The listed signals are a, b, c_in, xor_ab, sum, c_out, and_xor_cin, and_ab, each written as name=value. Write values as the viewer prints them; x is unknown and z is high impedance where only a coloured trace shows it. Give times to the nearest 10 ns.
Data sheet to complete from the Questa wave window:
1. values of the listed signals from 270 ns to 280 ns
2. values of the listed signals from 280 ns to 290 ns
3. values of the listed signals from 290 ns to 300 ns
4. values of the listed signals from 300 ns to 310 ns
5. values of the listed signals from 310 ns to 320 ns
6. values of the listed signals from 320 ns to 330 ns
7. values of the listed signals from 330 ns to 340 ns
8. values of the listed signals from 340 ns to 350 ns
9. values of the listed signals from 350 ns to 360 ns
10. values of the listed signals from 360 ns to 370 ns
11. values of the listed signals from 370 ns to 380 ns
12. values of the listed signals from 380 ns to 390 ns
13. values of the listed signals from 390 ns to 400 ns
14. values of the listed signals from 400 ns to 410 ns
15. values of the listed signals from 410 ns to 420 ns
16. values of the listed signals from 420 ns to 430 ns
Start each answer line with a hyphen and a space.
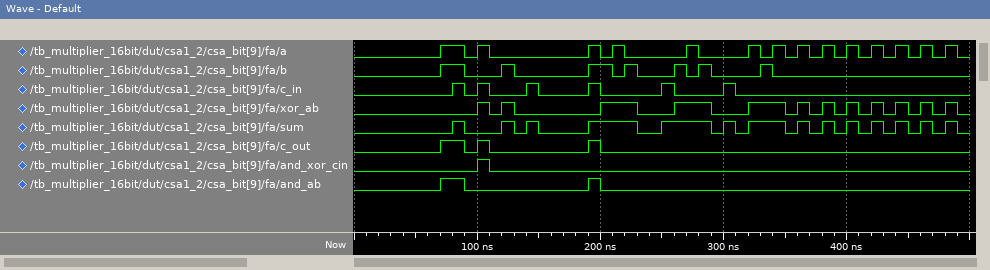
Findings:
- a=1, b=0, c_in=0, xor_ab=1, sum=1, c_out=0, and_xor_cin=0, and_ab=0
- a=0, b=1, c_in=0, xor_ab=1, sum=1, c_out=0, and_xor_cin=0, and_ab=0
- a=0, b=0, c_in=0, xor_ab=0, sum=0, c_out=0, and_xor_cin=0, and_ab=0
- a=0, b=0, c_in=1, xor_ab=0, sum=1, c_out=0, and_xor_cin=0, and_ab=0
- a=0, b=0, c_in=0, xor_ab=0, sum=0, c_out=0, and_xor_cin=0, and_ab=0
- a=1, b=0, c_in=0, xor_ab=1, sum=1, c_out=0, and_xor_cin=0, and_ab=0
- a=0, b=1, c_in=0, xor_ab=1, sum=1, c_out=0, and_xor_cin=0, and_ab=0
- a=1, b=0, c_in=0, xor_ab=1, sum=1, c_out=0, and_xor_cin=0, and_ab=0
- a=0, b=0, c_in=0, xor_ab=0, sum=0, c_out=0, and_xor_cin=0, and_ab=0
- a=1, b=0, c_in=0, xor_ab=1, sum=1, c_out=0, and_xor_cin=0, and_ab=0
- a=0, b=0, c_in=0, xor_ab=0, sum=0, c_out=0, and_xor_cin=0, and_ab=0
- a=1, b=0, c_in=0, xor_ab=1, sum=1, c_out=0, and_xor_cin=0, and_ab=0
- a=0, b=0, c_in=0, xor_ab=0, sum=0, c_out=0, and_xor_cin=0, and_ab=0
- a=1, b=0, c_in=0, xor_ab=1, sum=1, c_out=0, and_xor_cin=0, and_ab=0
- a=0, b=0, c_in=0, xor_ab=0, sum=0, c_out=0, and_xor_cin=0, and_ab=0
- a=1, b=0, c_in=0, xor_ab=1, sum=1, c_out=0, and_xor_cin=0, and_ab=0
